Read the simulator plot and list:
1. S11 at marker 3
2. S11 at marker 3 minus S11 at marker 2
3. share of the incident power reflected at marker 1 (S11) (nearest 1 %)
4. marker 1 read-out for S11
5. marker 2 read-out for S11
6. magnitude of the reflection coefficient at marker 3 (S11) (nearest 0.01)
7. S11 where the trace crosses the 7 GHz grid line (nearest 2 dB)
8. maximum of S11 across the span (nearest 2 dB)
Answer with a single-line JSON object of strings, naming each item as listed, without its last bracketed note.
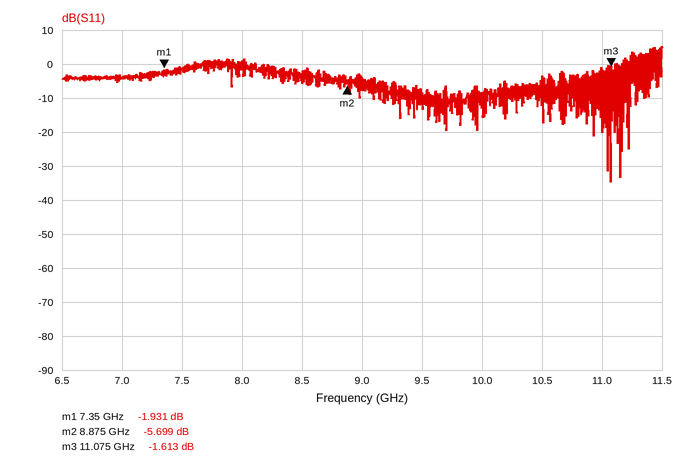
{"S11 at marker 3": "-1.613 dB", "S11 at marker 3 minus S11 at marker 2": "4.086 dB", "share of the incident power reflected at marker 1 (S11)": "64 %", "marker 1 read-out for S11": "-1.931 dB", "marker 2 read-out for S11": "-5.699 dB", "magnitude of the reflection coefficient at marker 3 (S11)": "0.83", "S11 where the trace crosses the 7 GHz grid line": "-4 dB", "maximum of S11 across the span": "6 dB"}
